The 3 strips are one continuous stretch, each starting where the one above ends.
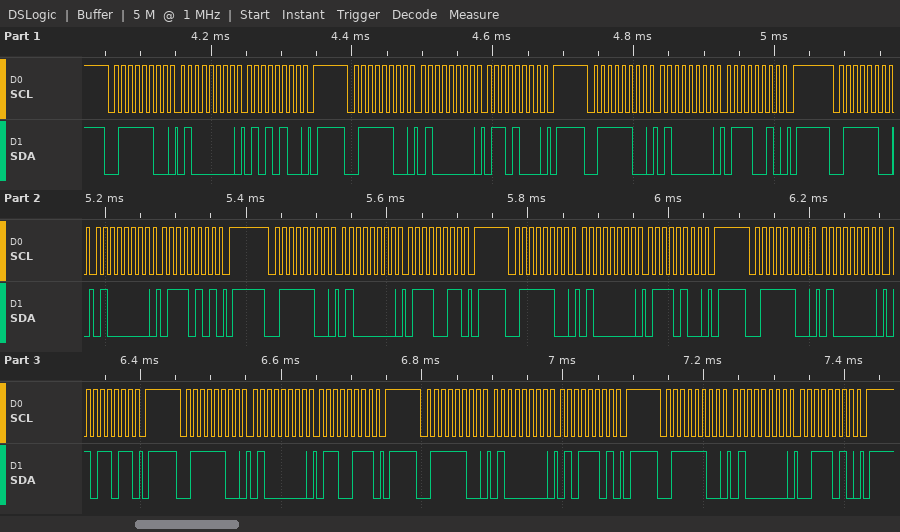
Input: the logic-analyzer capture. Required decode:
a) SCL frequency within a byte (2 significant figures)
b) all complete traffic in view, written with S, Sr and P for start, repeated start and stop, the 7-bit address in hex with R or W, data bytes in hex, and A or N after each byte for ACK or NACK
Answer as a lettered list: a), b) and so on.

a) 100 kHz
b) S 3EW A 40 A 54 A P S 3EW A 40 A 68 A P S 3EW A 40 A 72 A P S 3EW A 40 A 75 A P S 3EW A 40 A 73 A P S 3EW A 40 A 74 A P S 3EW A 40 A 5B A P S 3EW A 40 A 67 A P S 3EW A 40 A 5D A P S 3EW A 40 A 3A A P
